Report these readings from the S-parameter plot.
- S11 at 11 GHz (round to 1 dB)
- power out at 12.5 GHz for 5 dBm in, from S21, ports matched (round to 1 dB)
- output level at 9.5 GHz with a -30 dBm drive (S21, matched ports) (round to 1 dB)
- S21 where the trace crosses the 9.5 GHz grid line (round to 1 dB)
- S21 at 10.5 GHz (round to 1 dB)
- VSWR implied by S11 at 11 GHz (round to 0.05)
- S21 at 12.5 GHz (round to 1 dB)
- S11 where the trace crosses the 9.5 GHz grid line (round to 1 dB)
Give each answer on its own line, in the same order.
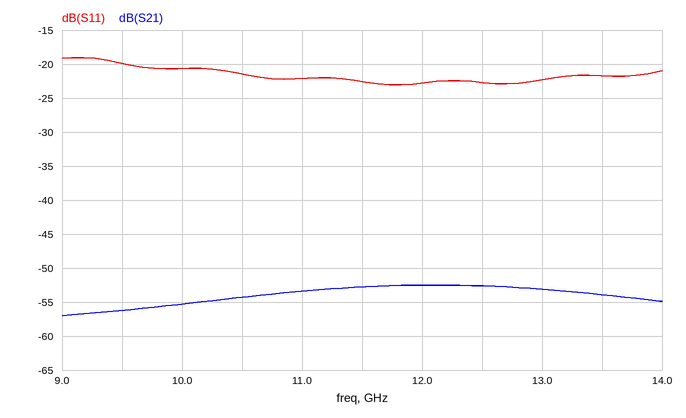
-22 dB
-48 dBm
-86 dBm
-56 dB
-54 dB
1.15
-53 dB
-20 dB
